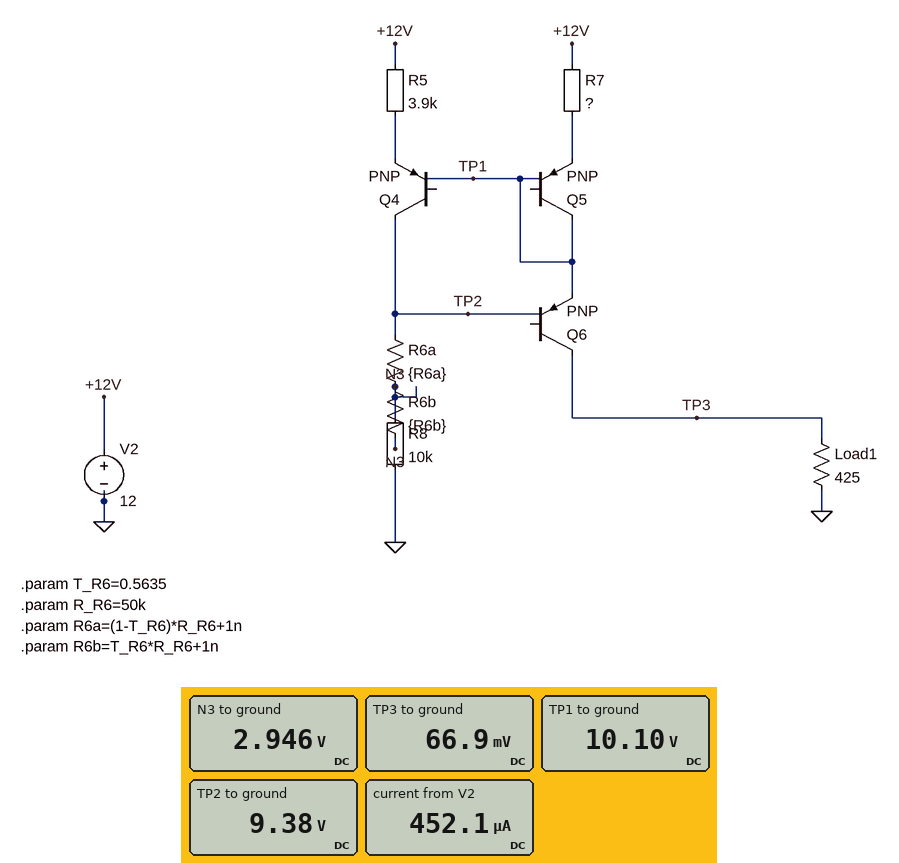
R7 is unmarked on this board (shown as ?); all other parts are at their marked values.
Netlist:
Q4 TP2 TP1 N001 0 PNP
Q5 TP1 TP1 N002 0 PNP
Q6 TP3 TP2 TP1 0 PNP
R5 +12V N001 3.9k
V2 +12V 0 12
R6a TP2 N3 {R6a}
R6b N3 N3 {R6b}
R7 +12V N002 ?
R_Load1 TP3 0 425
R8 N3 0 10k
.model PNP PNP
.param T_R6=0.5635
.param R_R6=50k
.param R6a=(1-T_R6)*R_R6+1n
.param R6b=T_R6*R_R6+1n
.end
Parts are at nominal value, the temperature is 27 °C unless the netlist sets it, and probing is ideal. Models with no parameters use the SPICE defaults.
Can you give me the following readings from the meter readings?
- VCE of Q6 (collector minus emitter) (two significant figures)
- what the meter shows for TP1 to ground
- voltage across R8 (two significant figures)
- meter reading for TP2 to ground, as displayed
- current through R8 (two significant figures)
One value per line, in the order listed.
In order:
-10 V
10.10 V
2.9 V
9.38 V
290 µA
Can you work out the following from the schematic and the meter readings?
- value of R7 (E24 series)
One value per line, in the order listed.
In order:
7.5 kΩ
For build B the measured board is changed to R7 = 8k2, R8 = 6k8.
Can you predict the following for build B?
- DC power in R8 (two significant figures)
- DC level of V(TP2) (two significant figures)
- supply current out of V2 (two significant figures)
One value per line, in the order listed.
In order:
710 µW
9.3 V
480 µA
